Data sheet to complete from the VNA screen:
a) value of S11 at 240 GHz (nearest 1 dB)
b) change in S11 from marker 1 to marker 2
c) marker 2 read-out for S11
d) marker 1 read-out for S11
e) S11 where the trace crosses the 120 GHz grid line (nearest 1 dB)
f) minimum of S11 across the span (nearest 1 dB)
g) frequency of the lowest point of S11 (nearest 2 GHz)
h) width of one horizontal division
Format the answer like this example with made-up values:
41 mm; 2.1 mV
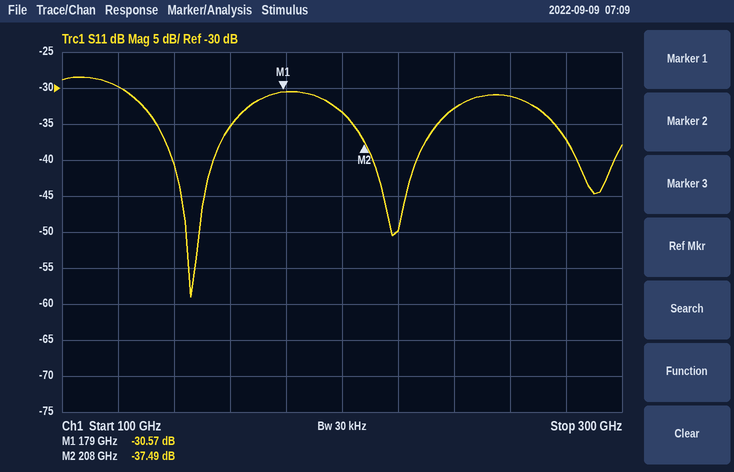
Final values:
-33 dB; -6.92 dB; -37.49 dB; -30.57 dB; -30 dB; -59 dB; 146 GHz; 20 GHz
